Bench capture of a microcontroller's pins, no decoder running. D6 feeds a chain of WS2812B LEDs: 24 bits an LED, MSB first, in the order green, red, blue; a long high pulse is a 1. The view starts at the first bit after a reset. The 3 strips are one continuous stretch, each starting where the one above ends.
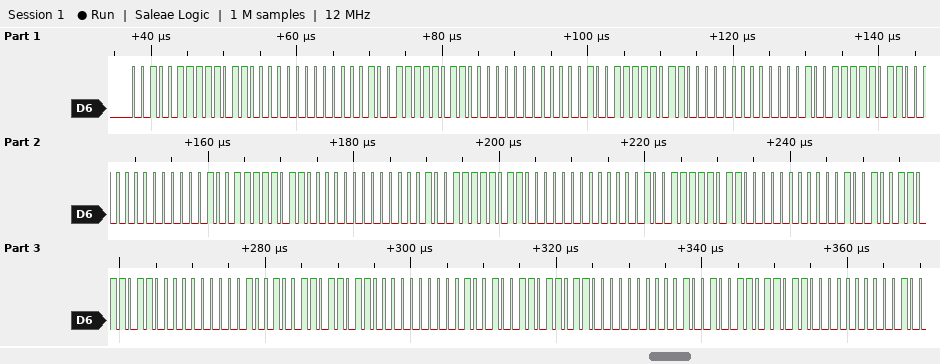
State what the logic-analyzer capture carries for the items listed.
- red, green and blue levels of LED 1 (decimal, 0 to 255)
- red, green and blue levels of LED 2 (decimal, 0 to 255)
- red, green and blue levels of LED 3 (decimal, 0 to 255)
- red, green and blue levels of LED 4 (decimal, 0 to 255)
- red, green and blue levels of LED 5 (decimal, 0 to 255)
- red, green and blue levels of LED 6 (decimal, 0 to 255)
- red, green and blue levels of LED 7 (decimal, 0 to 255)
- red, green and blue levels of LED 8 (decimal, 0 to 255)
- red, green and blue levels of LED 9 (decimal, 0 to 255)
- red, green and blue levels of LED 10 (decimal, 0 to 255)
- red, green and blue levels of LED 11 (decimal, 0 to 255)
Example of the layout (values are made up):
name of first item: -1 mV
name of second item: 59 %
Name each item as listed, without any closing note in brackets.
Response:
red, green and blue levels of LED 1: 216, 39, 0
red, green and blue levels of LED 2: 216, 39, 0
red, green and blue levels of LED 3: 216, 39, 0
red, green and blue levels of LED 4: 216, 39, 0
red, green and blue levels of LED 5: 216, 39, 0
red, green and blue levels of LED 6: 216, 39, 0
red, green and blue levels of LED 7: 216, 39, 0
red, green and blue levels of LED 8: 108, 147, 0
red, green and blue levels of LED 9: 108, 147, 0
red, green and blue levels of LED 10: 108, 147, 0
red, green and blue levels of LED 11: 108, 147, 0
